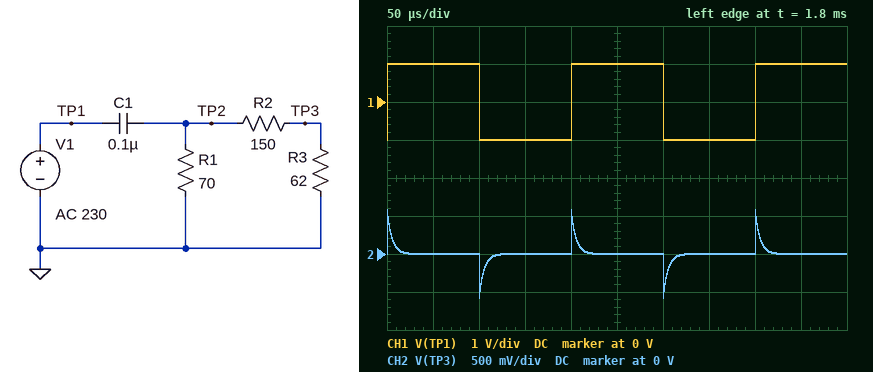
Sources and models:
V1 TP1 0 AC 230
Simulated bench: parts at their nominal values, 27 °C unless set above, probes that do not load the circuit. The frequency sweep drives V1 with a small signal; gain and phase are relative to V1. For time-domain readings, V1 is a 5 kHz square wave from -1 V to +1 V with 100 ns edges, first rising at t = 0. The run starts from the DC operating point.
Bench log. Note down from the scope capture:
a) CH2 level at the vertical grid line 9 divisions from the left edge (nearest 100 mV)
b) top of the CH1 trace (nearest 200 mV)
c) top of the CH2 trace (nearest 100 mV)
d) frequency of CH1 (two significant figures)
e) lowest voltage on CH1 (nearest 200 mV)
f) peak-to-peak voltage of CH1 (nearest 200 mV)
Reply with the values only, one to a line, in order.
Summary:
0 V
1.0 V
600 mV
5.0 kHz
-1.0 V
2.0 V
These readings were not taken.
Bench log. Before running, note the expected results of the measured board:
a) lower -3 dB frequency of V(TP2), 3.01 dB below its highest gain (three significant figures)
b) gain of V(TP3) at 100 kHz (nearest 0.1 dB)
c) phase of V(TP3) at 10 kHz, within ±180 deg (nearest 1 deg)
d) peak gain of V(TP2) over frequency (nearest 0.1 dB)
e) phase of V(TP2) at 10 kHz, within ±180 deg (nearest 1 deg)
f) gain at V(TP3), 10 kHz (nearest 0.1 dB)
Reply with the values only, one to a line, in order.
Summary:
30.2 kHz
-11.1 dB
72 deg
0 dB
72 deg
-20.7 dB
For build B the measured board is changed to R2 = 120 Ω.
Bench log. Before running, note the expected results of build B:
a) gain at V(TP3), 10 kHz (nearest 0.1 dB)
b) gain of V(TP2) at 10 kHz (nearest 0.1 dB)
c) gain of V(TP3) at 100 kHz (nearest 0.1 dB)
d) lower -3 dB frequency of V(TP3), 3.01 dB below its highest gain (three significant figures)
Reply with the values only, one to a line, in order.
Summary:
-19.7 dB
-10.4 dB
-9.8 dB
31.5 kHz
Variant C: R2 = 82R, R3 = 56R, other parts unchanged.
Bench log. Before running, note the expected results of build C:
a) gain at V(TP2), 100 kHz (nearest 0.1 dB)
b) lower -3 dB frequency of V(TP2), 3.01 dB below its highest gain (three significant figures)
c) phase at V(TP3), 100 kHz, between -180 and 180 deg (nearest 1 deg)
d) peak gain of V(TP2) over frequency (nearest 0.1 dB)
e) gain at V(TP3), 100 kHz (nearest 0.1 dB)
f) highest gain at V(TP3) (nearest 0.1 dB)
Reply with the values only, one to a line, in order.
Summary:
-0.5 dB
34.3 kHz
19 deg
0 dB
-8.3 dB
-7.8 dB
